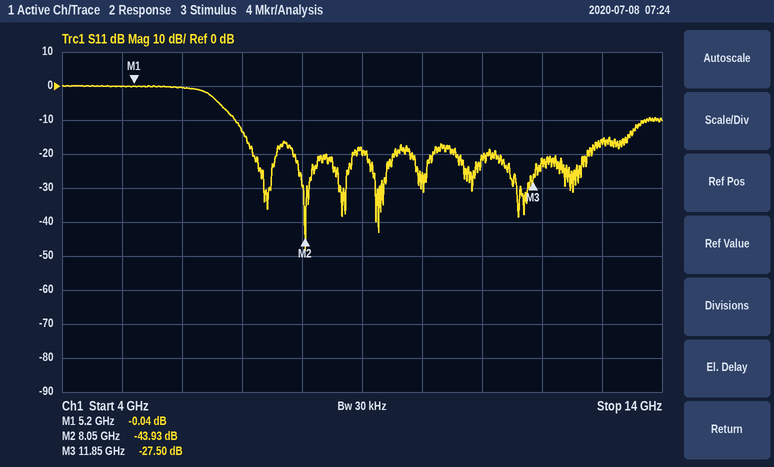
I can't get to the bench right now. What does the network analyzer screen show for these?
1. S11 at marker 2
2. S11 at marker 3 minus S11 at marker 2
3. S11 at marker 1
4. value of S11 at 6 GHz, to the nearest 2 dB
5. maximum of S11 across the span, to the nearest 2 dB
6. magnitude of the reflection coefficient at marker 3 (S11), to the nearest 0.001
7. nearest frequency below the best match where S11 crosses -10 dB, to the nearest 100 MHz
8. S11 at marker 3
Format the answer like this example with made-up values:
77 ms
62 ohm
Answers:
-43.93 dB
16.43 dB
-0.04 dB
0 dB
0 dB
0.042
6.9 GHz
-27.50 dB
